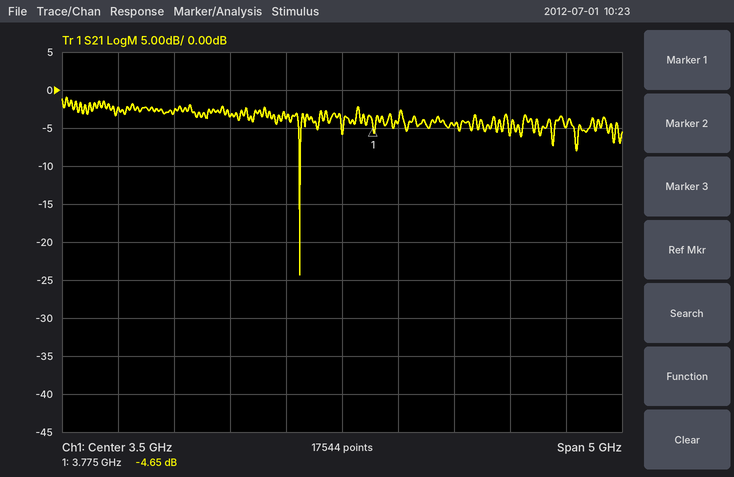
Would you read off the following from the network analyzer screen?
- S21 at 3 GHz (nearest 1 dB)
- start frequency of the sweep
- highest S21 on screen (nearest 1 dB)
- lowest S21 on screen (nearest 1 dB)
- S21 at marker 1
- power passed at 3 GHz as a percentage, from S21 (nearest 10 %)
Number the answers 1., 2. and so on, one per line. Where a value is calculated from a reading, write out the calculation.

1. -4 dB
2. 1 GHz
3. -1 dB
4. -24 dB
5. -4.65 dB
6. 10^(-4/10) ≈ 40 %
